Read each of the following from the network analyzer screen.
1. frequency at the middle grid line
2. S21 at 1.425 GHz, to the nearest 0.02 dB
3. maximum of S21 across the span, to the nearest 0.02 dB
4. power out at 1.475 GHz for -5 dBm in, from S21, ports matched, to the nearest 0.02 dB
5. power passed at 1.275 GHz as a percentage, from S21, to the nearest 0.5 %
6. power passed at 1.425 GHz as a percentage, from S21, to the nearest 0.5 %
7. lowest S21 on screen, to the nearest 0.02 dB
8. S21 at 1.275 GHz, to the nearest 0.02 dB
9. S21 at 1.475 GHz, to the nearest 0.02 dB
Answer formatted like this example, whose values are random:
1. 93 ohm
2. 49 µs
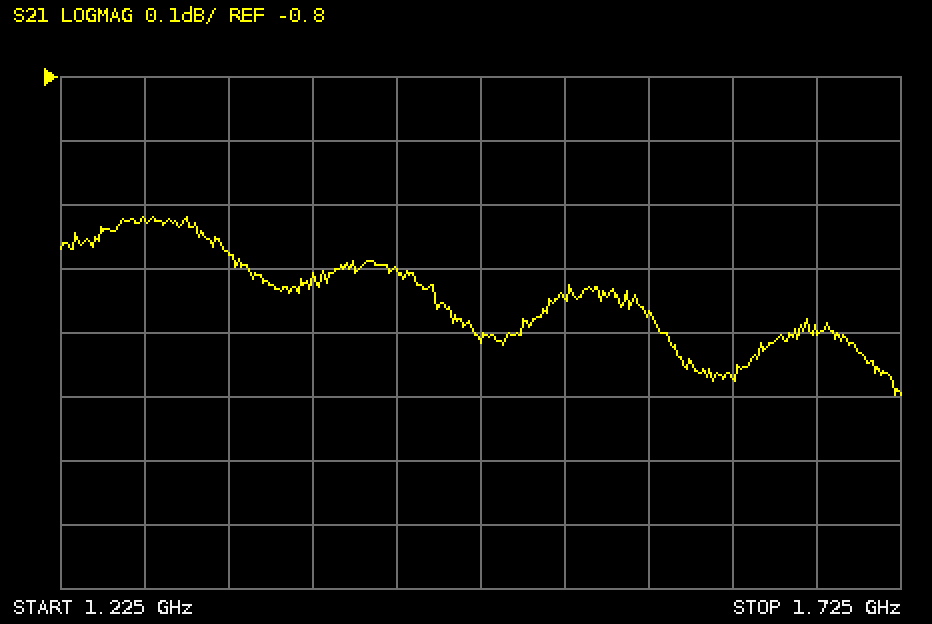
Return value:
1. 1.475 GHz
2. -1.10 dB
3. -1.02 dB
4. -6.22 dBm
5. 79.0 %
6. 77.5 %
7. -1.30 dB
8. -1.02 dB
9. -1.22 dB
